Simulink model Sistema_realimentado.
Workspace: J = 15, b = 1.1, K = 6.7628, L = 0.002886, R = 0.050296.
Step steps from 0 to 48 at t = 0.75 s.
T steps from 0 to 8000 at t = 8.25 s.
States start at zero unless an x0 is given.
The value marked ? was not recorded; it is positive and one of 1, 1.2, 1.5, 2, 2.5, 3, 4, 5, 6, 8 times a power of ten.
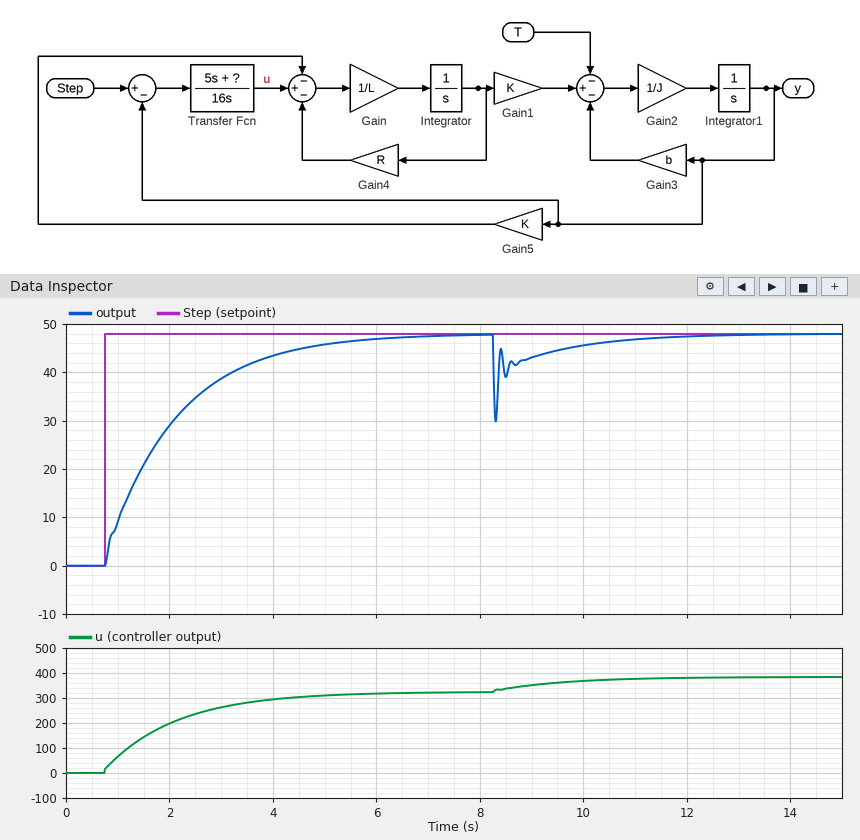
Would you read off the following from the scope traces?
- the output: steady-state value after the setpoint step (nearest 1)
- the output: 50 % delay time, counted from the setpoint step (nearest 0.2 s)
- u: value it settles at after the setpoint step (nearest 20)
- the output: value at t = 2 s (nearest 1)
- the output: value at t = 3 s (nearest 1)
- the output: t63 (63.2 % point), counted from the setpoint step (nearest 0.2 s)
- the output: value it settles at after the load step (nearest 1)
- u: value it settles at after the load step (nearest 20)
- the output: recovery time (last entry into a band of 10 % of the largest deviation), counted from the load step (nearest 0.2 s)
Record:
48
1.0 s
320
29
39
1.4 s
48
380
2.2 s
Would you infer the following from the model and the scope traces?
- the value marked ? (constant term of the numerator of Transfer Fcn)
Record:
80
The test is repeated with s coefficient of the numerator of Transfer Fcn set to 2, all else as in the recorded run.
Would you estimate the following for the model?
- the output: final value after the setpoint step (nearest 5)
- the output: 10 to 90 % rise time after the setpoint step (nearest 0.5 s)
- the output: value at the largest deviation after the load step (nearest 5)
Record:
50
3.0 s
30
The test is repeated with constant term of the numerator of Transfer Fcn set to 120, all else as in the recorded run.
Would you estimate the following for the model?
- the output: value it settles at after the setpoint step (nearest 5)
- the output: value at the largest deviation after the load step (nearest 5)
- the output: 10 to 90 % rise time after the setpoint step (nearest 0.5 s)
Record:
50
30
2.0 s
